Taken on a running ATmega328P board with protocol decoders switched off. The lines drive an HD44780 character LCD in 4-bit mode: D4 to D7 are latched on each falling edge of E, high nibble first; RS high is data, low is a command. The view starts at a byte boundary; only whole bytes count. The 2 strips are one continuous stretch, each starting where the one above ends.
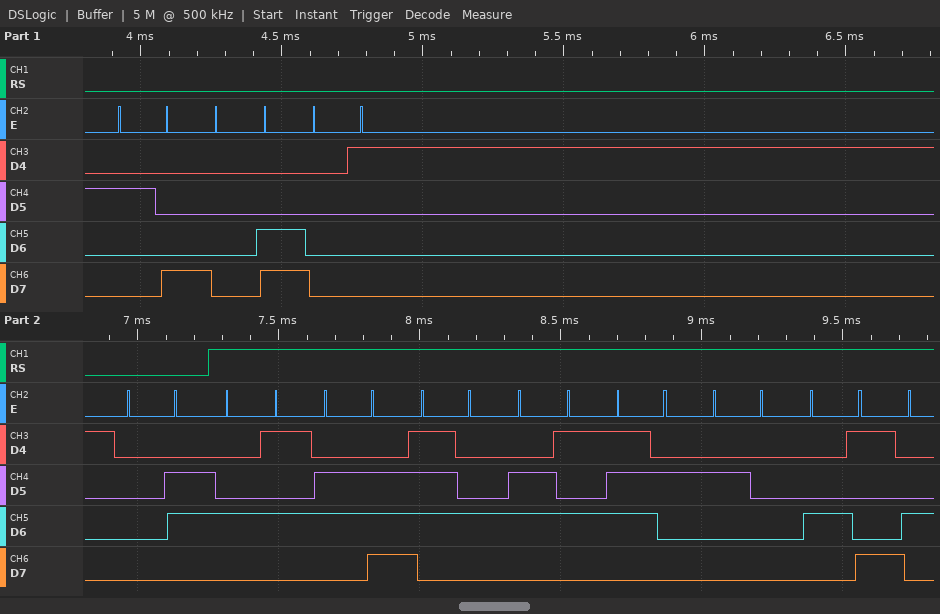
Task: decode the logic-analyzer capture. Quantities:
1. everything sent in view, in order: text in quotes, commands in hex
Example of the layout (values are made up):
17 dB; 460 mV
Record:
0x28 0x0C 0x01 0x06 "Enter I"
